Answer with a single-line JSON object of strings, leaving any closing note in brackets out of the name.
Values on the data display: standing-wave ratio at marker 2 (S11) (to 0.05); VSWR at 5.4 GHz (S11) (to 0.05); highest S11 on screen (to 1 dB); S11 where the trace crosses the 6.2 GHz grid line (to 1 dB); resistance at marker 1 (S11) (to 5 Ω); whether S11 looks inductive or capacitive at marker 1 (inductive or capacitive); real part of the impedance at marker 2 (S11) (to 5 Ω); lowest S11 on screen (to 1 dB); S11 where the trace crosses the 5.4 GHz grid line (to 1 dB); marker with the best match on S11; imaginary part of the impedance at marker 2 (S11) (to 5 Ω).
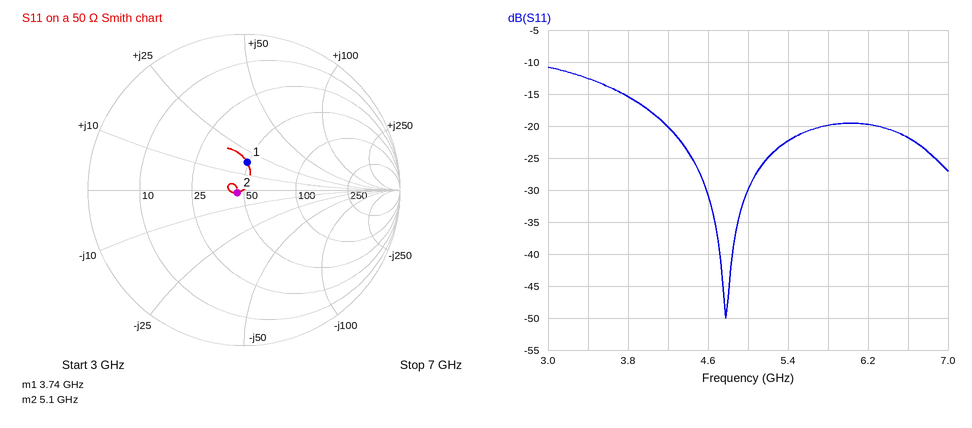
{"standing-wave ratio at marker 2 (S11)": "1.10", "VSWR at 5.4 GHz (S11)": "1.15", "highest S11 on screen": "-11 dB", "S11 where the trace crosses the 6.2 GHz grid line": "-20 dB", "resistance at marker 1 (S11)": "50 Ω", "whether S11 looks inductive or capacitive at marker 1": "inductive", "real part of the impedance at marker 2 (S11)": "45 Ω", "lowest S11 on screen": "-50 dB", "S11 where the trace crosses the 5.4 GHz grid line": "-22 dB", "marker with the best match on S11": "marker 2", "imaginary part of the impedance at marker 2 (S11)": "0 Ω"}
